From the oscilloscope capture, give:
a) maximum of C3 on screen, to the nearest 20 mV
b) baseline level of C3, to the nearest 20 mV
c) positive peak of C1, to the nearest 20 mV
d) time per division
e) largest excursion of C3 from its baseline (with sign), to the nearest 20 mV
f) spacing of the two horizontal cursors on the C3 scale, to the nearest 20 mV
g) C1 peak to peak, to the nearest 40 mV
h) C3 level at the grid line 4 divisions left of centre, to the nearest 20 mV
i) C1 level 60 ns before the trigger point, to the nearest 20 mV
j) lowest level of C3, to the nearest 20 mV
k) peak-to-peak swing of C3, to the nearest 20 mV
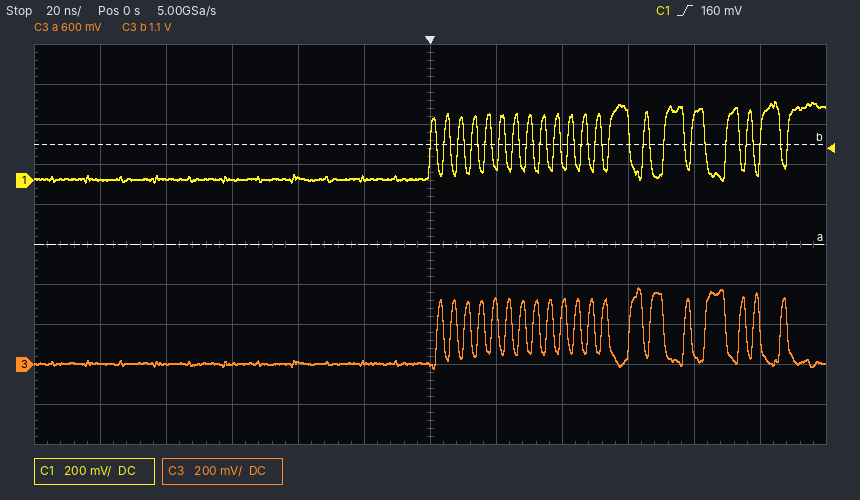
380 mV
0 mV
400 mV
20 ns
+380 mV
500 mV
400 mV
0 mV
0 mV
-20 mV
400 mV
